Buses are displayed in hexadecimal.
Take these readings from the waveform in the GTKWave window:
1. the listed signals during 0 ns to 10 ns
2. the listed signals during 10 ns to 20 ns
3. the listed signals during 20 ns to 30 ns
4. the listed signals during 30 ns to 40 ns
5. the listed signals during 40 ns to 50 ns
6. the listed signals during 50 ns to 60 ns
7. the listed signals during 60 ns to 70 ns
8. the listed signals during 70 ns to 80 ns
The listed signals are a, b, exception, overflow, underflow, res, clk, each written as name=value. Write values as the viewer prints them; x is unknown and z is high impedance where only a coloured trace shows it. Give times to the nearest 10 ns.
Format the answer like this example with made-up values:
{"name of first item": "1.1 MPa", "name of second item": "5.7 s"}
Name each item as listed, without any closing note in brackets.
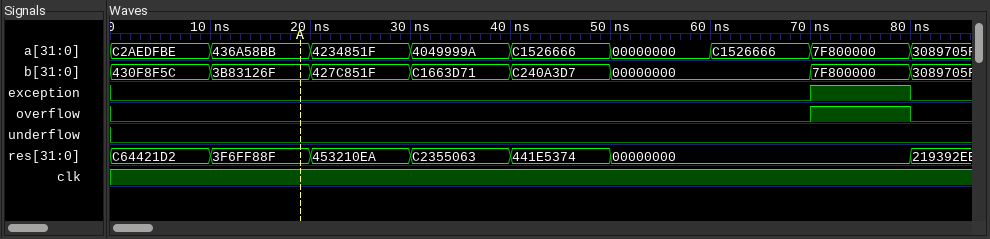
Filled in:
{"the listed signals during 0 ns to 10 ns": "a=C2AEDFBE, b=430F8F5C, exception=0, overflow=0, underflow=0, res=C64421D2, clk=1", "the listed signals during 10 ns to 20 ns": "a=436A58BB, b=3B83126F, exception=0, overflow=0, underflow=0, res=3F6FF88F, clk=1", "the listed signals during 20 ns to 30 ns": "a=4234851F, b=427C851F, exception=0, overflow=0, underflow=0, res=453210EA, clk=1", "the listed signals during 30 ns to 40 ns": "a=4049999A, b=C1663D71, exception=0, overflow=0, underflow=0, res=C2355063, clk=1", "the listed signals during 40 ns to 50 ns": "a=C1526666, b=C240A3D7, exception=0, overflow=0, underflow=0, res=441E5374, clk=1", "the listed signals during 50 ns to 60 ns": "a=00000000, b=00000000, exception=0, overflow=0, underflow=0, res=00000000, clk=1", "the listed signals during 60 ns to 70 ns": "a=C1526666, b=00000000, exception=0, overflow=0, underflow=0, res=00000000, clk=1", "the listed signals during 70 ns to 80 ns": "a=7F800000, b=7F800000, exception=1, overflow=1, underflow=0, res=00000000, clk=1"}
